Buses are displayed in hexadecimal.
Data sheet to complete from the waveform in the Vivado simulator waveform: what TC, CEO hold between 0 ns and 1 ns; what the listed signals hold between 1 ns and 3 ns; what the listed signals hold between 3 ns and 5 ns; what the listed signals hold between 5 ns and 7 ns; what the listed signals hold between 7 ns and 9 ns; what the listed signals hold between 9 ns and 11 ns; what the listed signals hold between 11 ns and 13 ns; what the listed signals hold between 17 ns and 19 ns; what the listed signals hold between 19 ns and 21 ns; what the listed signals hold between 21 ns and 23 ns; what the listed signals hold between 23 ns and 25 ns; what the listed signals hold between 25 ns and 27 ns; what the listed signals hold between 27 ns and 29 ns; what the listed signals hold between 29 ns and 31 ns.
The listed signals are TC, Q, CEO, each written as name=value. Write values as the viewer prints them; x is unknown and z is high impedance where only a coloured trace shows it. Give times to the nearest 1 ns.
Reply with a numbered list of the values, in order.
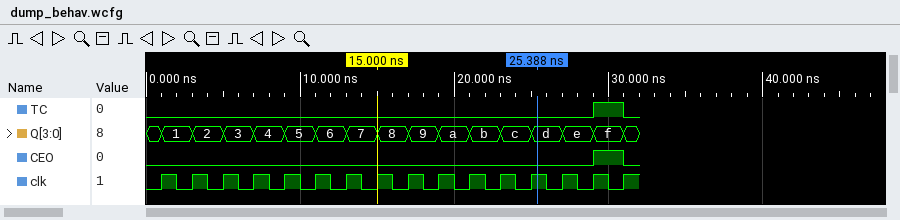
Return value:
1. TC=0, CEO=0
2. TC=0, Q=1, CEO=0
3. TC=0, Q=2, CEO=0
4. TC=0, Q=3, CEO=0
5. TC=0, Q=4, CEO=0
6. TC=0, Q=5, CEO=0
7. TC=0, Q=6, CEO=0
8. TC=0, Q=9, CEO=0
9. TC=0, Q=a, CEO=0
10. TC=0, Q=b, CEO=0
11. TC=0, Q=c, CEO=0
12. TC=0, Q=d, CEO=0
13. TC=0, Q=e, CEO=0
14. TC=1, Q=f, CEO=1
